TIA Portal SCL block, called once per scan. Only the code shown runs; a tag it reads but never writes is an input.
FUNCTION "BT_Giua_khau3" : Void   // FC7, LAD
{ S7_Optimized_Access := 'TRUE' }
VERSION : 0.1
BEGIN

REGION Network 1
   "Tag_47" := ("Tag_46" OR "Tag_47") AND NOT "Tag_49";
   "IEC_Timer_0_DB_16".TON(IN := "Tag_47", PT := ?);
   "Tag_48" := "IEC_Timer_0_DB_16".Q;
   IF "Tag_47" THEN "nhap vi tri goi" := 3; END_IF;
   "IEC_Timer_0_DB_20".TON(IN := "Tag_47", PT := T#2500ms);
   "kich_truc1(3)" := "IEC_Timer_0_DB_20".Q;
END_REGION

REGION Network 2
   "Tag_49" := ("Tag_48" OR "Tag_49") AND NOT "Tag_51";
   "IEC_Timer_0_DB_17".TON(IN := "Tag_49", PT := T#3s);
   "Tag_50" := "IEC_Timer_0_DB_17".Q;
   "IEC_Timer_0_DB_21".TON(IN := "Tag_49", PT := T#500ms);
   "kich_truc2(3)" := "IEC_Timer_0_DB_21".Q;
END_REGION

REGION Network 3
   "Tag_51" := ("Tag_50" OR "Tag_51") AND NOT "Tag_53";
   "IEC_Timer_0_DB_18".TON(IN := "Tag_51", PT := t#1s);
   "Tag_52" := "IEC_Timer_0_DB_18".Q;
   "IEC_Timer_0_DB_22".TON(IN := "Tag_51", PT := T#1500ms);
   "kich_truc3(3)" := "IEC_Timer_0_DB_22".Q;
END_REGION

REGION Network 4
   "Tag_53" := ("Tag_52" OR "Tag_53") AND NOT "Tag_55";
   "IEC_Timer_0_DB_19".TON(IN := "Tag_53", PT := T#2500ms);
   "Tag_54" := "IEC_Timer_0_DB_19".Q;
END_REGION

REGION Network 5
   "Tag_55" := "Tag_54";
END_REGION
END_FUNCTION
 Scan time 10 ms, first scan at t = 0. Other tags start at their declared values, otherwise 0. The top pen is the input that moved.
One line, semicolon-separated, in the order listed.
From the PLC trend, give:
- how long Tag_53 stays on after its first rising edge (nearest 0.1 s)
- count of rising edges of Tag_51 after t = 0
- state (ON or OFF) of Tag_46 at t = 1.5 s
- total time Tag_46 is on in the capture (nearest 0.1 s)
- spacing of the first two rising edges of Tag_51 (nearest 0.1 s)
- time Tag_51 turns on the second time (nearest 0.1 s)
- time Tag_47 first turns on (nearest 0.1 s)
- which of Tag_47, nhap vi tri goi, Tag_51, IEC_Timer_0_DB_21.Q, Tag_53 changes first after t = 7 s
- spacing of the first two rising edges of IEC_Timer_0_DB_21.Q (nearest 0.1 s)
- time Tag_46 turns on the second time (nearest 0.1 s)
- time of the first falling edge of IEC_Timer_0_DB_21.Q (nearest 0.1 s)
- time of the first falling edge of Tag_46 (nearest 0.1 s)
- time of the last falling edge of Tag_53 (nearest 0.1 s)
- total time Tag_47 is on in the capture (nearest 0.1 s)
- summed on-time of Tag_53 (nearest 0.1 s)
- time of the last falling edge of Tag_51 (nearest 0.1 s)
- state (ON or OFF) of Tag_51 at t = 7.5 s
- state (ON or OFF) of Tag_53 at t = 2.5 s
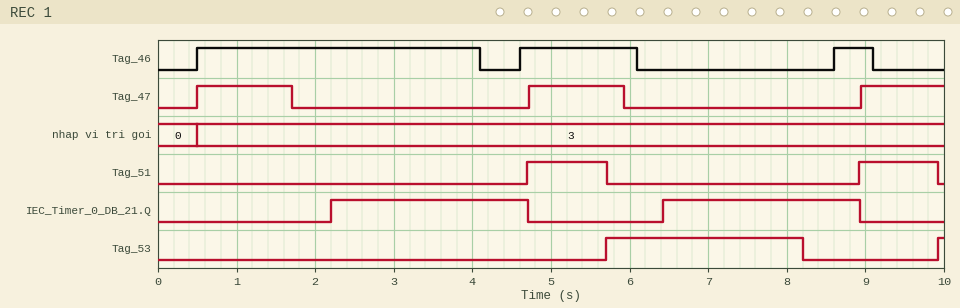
2.5 s; 2; ON; 5.6 s; 4.2 s; 8.9 s; 0.5 s; Tag_53; 4.2 s; 4.6 s; 4.7 s; 4.1 s; 8.2 s; 3.5 s; 2.6 s; 9.9 s; OFF; OFF
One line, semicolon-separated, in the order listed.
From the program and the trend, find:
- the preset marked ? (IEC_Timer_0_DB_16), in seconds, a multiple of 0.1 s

1.2 s
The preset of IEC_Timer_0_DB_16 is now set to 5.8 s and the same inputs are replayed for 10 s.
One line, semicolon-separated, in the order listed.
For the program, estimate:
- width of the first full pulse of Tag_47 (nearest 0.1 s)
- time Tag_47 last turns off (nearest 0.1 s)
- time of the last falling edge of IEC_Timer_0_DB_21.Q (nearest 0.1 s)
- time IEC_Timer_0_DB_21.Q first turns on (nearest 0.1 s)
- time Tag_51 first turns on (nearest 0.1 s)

5.8 s; 6.3 s; 9.3 s; 6.8 s; 9.3 s
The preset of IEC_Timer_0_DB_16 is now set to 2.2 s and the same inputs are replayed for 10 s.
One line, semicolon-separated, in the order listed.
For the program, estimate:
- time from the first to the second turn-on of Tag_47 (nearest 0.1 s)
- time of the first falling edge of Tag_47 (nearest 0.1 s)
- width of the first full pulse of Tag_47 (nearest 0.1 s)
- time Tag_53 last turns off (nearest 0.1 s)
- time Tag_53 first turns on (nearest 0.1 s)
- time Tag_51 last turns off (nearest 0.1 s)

5.2 s; 2.7 s; 2.2 s; 9.2 s; 6.7 s; 6.7 s
